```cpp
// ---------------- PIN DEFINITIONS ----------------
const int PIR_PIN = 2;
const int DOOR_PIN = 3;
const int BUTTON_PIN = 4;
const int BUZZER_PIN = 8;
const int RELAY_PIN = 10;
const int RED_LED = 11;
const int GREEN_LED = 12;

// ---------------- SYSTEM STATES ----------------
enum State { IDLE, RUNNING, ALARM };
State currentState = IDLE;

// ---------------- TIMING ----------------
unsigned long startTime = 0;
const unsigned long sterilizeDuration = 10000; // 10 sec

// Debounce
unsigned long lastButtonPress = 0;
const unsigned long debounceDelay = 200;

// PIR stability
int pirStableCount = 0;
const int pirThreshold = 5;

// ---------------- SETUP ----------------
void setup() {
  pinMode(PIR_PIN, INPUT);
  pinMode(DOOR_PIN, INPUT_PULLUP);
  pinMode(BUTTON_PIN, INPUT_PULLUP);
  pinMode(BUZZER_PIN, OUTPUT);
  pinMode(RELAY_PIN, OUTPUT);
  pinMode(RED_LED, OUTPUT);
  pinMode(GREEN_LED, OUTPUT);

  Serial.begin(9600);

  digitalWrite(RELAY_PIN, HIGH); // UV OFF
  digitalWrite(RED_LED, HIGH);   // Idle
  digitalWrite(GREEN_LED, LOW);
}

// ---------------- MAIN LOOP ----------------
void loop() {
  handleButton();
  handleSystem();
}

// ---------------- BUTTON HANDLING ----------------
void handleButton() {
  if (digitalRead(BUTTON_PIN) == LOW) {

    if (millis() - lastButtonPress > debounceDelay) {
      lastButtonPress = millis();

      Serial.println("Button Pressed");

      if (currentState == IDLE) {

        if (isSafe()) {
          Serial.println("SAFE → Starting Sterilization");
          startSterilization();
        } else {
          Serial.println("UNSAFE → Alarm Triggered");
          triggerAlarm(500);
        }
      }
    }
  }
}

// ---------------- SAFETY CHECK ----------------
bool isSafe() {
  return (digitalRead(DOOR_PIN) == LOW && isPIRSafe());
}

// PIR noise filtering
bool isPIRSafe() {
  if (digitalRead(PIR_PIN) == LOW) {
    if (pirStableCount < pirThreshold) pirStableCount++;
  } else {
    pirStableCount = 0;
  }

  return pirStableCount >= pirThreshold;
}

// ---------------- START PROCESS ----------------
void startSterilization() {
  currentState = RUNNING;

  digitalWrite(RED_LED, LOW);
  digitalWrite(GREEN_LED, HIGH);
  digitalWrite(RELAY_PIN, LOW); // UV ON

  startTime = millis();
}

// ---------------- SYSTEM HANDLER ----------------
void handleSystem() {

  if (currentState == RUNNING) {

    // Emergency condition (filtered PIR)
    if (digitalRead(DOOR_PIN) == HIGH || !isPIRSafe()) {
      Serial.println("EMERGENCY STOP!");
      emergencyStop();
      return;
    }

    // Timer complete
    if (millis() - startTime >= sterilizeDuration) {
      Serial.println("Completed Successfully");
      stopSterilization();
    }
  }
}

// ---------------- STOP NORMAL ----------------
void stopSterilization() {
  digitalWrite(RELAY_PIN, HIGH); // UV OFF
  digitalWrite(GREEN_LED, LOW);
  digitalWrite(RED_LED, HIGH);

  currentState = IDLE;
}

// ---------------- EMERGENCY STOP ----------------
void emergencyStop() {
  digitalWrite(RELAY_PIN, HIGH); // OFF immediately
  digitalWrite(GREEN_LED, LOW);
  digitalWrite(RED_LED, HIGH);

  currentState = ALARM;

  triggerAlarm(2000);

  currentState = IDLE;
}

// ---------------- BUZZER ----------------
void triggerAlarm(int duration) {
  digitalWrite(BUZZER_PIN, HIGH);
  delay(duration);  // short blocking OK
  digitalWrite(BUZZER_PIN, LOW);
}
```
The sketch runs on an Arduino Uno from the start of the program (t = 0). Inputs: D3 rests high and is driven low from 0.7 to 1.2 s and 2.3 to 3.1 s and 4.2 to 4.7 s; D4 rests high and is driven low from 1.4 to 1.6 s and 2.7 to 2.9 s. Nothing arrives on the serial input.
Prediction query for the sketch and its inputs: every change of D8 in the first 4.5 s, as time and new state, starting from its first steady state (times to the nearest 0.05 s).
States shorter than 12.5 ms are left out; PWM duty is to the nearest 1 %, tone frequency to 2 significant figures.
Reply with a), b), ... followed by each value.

a) 0 s low; 1.4 s high; 1.9 s low; 2.7 s high; 3.2 s low
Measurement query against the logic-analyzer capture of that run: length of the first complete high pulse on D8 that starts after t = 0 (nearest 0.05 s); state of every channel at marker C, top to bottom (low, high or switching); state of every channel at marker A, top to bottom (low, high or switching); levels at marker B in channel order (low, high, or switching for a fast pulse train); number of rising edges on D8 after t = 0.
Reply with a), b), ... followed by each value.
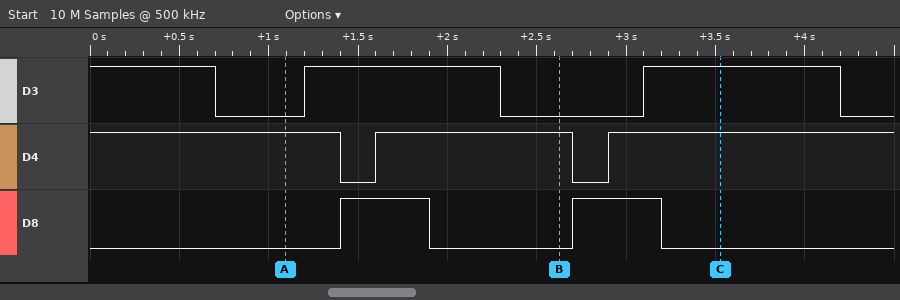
a) 0.50 s
b) D3 high, D4 high, D8 low
c) D3 low, D4 high, D8 low
d) D3 low, D4 high, D8 low
e) 2
